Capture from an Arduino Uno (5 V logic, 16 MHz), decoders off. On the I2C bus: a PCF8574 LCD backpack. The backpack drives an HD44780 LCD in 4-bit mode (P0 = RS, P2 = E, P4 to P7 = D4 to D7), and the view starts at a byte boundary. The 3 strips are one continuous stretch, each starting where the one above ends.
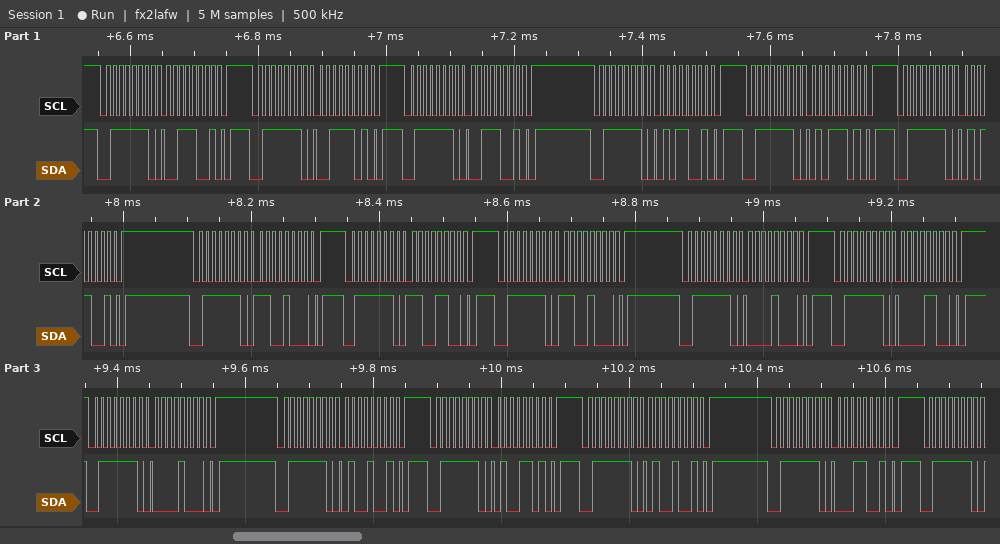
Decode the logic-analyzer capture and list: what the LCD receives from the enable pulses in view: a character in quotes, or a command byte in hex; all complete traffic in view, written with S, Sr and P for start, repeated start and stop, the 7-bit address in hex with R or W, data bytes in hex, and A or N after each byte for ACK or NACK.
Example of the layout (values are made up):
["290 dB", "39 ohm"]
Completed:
["'5' 0xC0", "S 3FW A 39 A P S 3FW A 3D A P S 3FW A 39 A P S 3FW A 59 A P S 3FW A 5D A P S 3FW A 59 A P S 3FW A C8 A P S 3FW A CC A P S 3FW A C8 A P S 3FW A 08 A P S 3FW A 0C A P S 3FW A 08 A P S 3FW A 49 A P S 3FW A 4D A P S 3FW A 49 A P S 3FW A 19 A P S 3FW A"]
